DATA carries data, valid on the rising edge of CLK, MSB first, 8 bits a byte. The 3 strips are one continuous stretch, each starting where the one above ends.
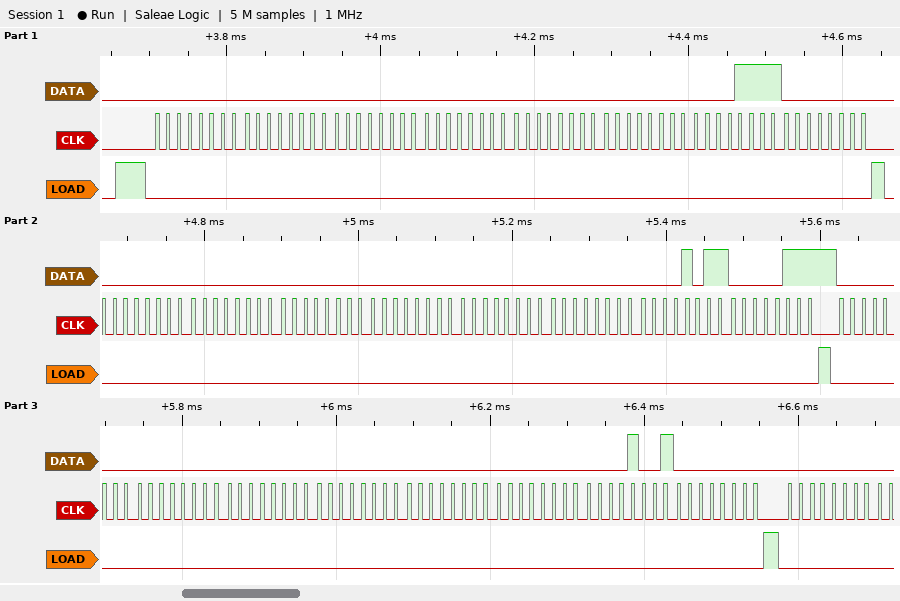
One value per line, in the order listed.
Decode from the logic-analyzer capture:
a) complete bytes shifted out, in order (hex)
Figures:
0x00 0x00 0x00 0x00 0x00 0x00 0x0F 0x00 0x00 0x00 0x00 0x00 0x00 0x00 0x0B 0x07 0x00 0x00 0x00 0x00 0x00 0x00 0x09 0x00 0x00
